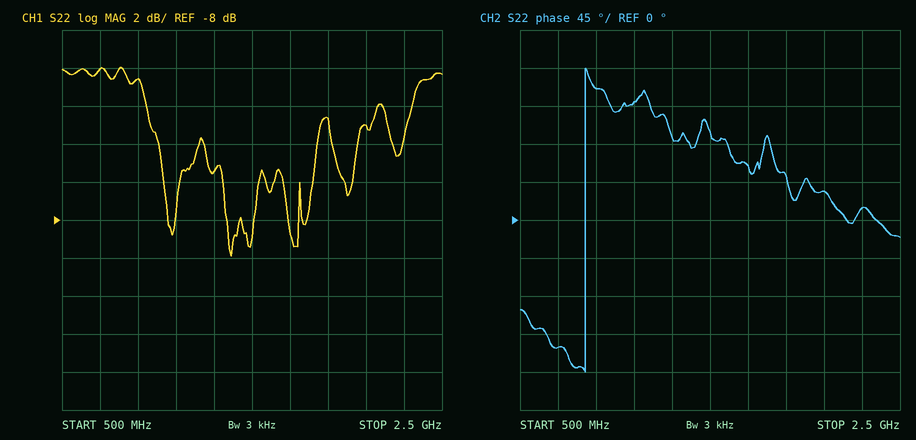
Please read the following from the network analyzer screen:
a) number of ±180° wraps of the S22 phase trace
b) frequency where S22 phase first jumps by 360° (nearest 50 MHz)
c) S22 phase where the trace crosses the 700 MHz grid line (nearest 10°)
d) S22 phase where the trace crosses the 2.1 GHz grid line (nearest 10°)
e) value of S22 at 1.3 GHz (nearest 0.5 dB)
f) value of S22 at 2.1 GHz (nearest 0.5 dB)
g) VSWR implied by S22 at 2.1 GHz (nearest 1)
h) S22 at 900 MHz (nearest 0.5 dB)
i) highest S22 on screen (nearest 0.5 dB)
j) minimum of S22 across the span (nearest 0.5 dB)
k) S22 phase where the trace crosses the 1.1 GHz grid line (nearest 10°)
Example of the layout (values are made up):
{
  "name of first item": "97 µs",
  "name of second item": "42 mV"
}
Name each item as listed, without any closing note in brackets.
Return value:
{
  "number of ±180° wraps of the S22 phase trace": "1",
  "frequency where S22 phase first jumps by 360°": "850 MHz",
  "S22 phase where the trace crosses the 700 MHz grid line": "-150°",
  "S22 phase where the trace crosses the 2.1 GHz grid line": "30°",
  "value of S22 at 1.3 GHz": "-5.5 dB",
  "value of S22 at 2.1 GHz": "-3.0 dB",
  "VSWR implied by S22 at 2.1 GHz": "6",
  "S22 at 900 MHz": "-0.5 dB",
  "highest S22 on screen": "0.0 dB",
  "minimum of S22 across the span": "-10.0 dB",
  "S22 phase where the trace crosses the 1.1 GHz grid line": "140°"
}
